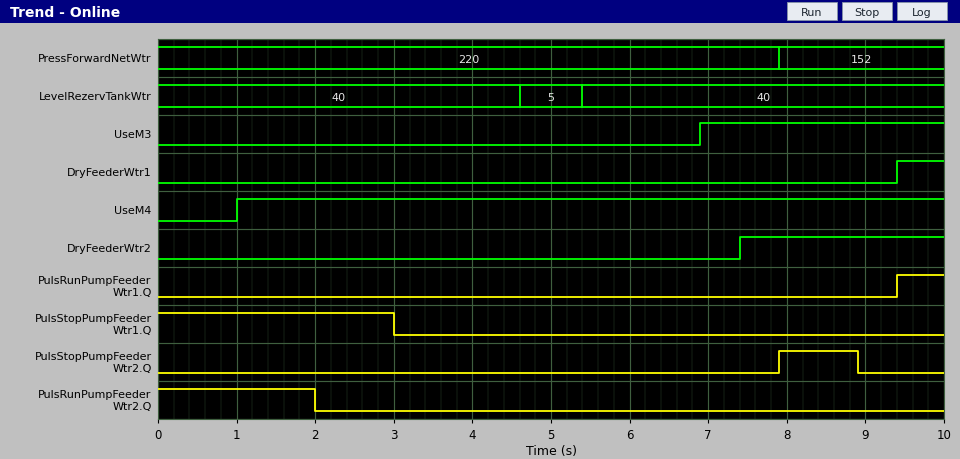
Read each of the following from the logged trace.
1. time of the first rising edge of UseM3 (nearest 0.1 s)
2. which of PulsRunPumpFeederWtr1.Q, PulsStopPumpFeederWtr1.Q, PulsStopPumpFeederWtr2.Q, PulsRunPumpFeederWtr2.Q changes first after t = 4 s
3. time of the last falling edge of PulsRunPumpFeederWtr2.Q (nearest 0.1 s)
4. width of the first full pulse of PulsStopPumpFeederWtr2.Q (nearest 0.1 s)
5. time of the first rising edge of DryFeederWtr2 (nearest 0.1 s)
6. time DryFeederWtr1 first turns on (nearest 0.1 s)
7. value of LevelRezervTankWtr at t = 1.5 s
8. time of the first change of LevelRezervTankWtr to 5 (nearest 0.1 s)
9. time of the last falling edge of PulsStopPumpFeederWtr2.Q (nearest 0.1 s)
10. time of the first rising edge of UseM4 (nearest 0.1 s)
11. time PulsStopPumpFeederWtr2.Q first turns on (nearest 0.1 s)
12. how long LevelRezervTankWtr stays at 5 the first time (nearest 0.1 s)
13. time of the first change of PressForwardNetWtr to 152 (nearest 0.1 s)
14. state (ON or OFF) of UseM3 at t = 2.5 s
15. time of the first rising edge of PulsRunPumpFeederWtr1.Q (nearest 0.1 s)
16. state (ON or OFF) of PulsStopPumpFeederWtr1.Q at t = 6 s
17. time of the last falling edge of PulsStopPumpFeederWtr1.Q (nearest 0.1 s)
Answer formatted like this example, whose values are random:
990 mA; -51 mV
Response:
6.9 s; PulsStopPumpFeederWtr2.Q; 2.0 s; 1.0 s; 7.4 s; 9.4 s; 40; 4.6 s; 8.9 s; 1.0 s; 7.9 s; 0.8 s; 7.9 s; OFF; 9.4 s; OFF; 3.0 s
